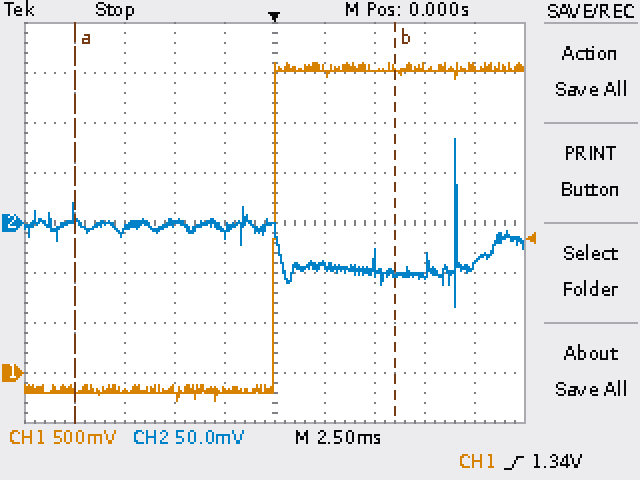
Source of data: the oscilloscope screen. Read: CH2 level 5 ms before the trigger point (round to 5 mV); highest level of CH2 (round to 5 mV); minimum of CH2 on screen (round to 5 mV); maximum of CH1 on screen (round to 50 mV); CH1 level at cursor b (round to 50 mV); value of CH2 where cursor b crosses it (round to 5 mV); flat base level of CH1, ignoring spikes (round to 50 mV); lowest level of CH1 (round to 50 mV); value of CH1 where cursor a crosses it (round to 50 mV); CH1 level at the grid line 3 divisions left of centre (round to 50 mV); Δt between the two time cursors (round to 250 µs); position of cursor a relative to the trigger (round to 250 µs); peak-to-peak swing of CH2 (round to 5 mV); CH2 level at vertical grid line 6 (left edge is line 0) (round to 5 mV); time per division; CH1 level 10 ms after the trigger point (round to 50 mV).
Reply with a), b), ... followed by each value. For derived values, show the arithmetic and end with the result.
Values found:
a) 0 mV
b) 85 mV
c) -85 mV
d) 3.10 V
e) 3.05 V
f) -50 mV
g) -200 mV
h) -300 mV
i) -150 mV
j) -200 mV
k) 16.00 ms
l) -10.00 ms
m) 85 mV − (-85 mV) = 170 mV
n) -45 mV
o) 2.5 ms
p) 3.05 V
